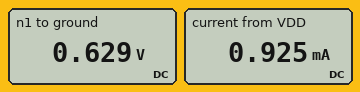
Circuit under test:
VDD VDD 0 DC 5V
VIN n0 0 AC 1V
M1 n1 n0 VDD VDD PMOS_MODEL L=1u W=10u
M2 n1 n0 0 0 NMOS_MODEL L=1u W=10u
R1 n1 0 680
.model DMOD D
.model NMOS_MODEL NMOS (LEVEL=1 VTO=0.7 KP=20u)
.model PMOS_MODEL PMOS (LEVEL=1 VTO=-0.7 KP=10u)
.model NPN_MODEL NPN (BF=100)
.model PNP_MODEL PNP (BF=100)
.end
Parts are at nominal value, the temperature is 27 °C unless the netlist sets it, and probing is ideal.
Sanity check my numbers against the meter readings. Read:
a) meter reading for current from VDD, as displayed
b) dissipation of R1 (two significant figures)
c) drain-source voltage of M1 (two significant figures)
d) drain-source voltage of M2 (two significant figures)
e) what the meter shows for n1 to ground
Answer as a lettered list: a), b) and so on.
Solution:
a) 0.925 mA
b) 580 µW
c) -4.4 V
d) 630 mV
e) 0.629 V
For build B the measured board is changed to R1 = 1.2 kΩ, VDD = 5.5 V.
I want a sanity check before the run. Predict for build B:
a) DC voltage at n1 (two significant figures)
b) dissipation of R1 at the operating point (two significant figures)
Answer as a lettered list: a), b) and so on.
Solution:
a) 1.4 V
b) 1.5 mW
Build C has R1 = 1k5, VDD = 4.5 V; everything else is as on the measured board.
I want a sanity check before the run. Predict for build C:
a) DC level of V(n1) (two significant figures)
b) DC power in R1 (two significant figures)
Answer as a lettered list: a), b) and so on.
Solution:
a) 1.1 V
b) 770 µW
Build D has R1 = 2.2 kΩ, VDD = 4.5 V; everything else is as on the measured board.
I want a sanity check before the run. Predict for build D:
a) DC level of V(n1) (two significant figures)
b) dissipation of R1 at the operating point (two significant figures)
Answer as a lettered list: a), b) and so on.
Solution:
a) 1.5 V
b) 1.0 mW
